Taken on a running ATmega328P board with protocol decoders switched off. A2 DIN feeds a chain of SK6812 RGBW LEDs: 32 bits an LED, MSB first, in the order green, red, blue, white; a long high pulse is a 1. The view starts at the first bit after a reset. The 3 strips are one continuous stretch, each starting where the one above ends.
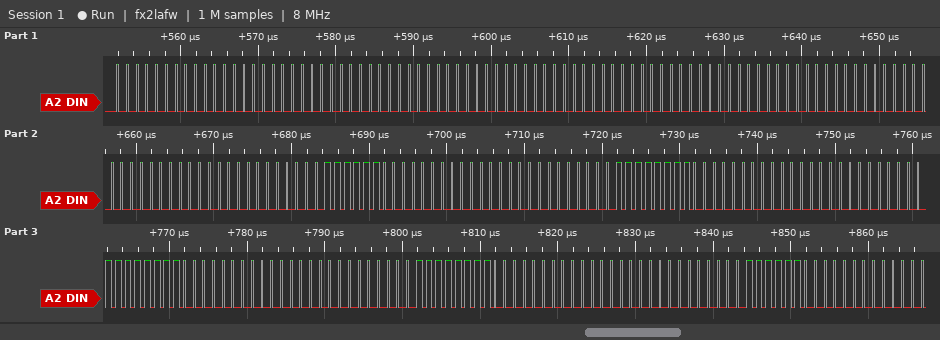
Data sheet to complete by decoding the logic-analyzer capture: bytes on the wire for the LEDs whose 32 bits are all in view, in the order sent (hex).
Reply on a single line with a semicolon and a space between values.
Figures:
00 00 00 00 00 00 00 00 00 00 00 00 00 3F 00 00 00 FF 00 00 00 FF 00 00 00 FF 00 00
